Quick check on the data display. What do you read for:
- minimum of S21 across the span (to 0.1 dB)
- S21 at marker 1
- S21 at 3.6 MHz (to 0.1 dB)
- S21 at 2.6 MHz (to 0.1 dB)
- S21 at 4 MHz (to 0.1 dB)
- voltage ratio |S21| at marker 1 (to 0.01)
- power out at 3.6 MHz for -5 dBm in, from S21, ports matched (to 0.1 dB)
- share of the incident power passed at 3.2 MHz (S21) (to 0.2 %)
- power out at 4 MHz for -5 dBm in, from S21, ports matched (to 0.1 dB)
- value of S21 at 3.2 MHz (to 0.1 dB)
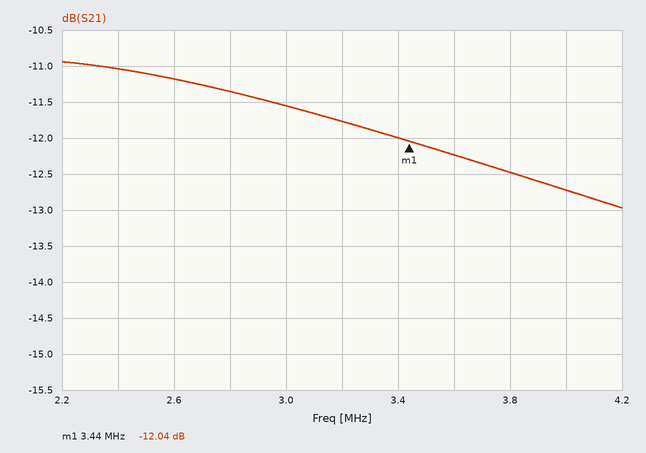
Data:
-13.0 dB
-12.04 dB
-12.2 dB
-11.2 dB
-12.7 dB
0.25
-17.2 dBm
6.6 %
-17.7 dBm
-11.8 dB
